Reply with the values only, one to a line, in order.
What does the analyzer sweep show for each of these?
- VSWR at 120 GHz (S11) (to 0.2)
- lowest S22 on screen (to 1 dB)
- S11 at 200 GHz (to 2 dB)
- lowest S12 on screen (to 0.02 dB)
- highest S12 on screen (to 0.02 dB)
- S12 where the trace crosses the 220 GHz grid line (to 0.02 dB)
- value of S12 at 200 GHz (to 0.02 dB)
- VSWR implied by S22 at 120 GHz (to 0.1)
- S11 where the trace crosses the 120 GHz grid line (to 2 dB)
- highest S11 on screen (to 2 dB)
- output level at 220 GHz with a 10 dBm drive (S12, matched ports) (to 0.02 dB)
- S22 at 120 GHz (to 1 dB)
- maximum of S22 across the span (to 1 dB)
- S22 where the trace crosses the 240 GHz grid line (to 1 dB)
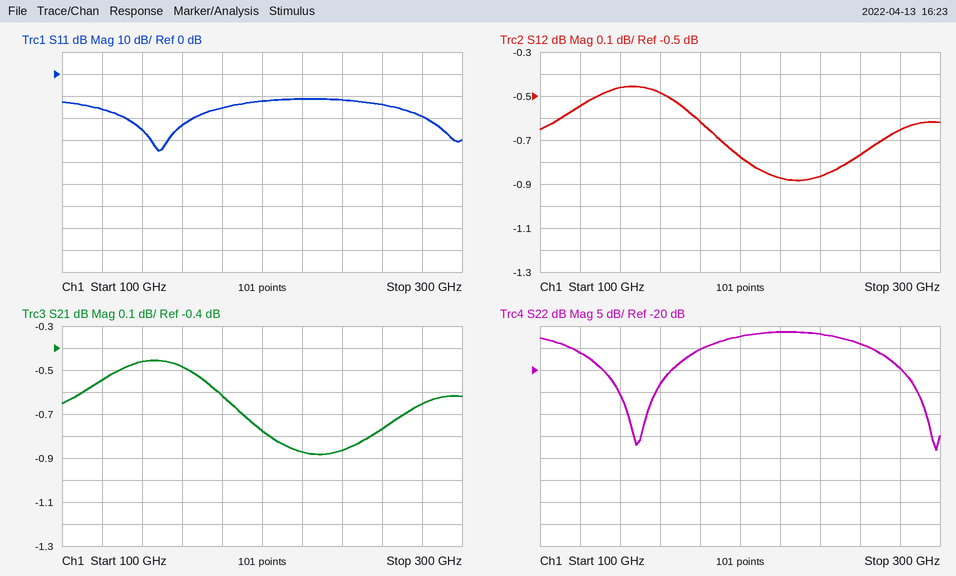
1.4
-38 dB
-12 dB
-0.88 dB
-0.46 dB
-0.88 dB
-0.78 dB
1.4
-16 dB
-12 dB
9.12 dBm
-16 dB
-11 dB
-12 dB
